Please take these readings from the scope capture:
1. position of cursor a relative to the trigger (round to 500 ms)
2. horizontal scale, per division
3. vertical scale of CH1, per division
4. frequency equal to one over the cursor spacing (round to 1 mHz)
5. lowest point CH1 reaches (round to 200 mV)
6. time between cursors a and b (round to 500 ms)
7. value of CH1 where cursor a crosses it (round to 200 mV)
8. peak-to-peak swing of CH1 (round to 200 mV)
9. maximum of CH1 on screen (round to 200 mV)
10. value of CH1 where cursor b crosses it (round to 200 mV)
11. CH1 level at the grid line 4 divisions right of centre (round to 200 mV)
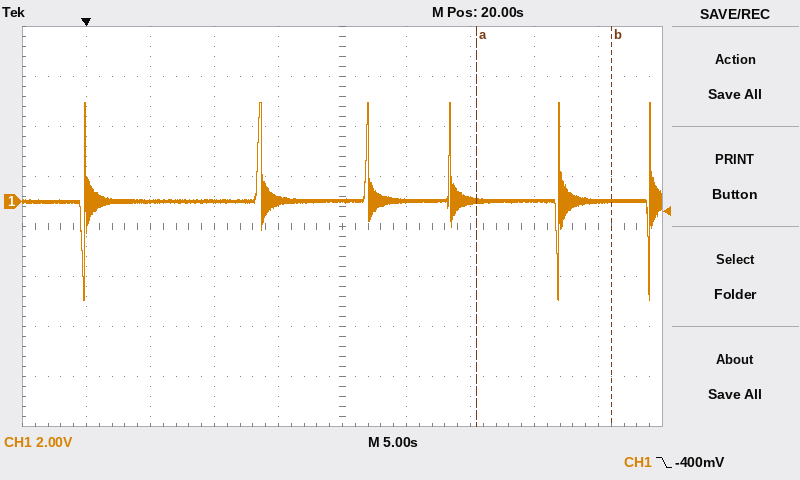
+30.5 s
5 s
2 V
95 mHz
-4.0 V
10.5 s
0.0 V
8.0 V
4.0 V
0.0 V
0.0 V
